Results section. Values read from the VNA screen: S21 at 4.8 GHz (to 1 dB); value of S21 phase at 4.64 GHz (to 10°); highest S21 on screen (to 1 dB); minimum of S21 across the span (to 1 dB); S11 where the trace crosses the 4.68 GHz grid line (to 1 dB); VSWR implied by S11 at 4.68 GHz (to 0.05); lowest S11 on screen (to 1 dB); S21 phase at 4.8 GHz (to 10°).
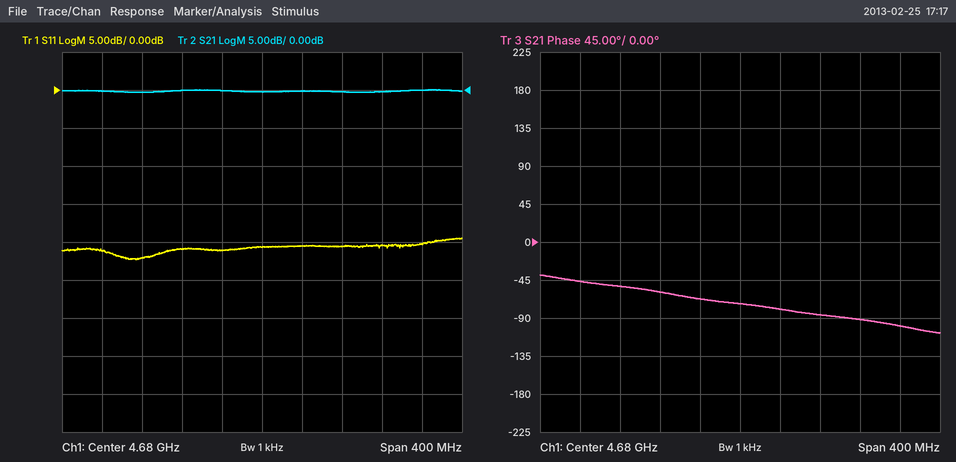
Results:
0 dB
-70°
0 dB
0 dB
-21 dB
1.20
-22 dB
-90°
